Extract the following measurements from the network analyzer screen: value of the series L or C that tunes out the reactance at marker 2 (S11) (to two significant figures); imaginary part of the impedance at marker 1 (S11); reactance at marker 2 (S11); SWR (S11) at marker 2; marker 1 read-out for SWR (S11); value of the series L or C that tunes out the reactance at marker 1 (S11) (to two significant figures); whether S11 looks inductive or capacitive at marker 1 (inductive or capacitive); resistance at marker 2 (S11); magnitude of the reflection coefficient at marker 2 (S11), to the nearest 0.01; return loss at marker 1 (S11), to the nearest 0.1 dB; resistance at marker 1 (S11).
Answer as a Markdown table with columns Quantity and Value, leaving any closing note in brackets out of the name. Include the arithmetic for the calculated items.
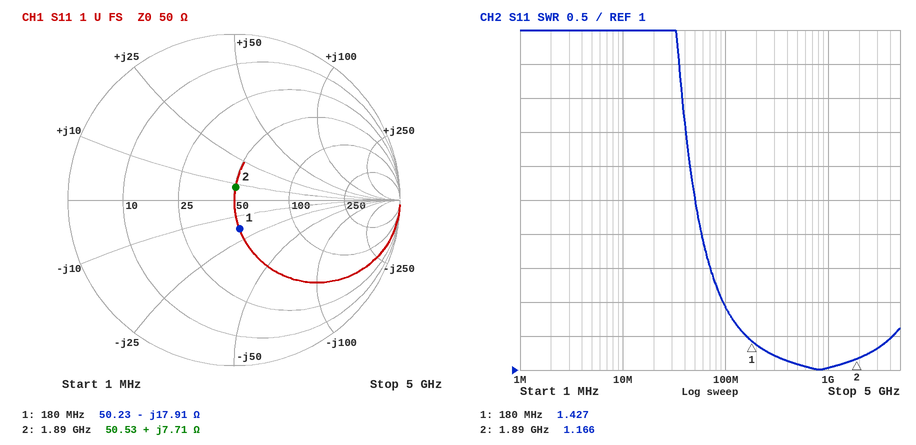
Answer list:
| Quantity | Value |
|---|---|
| value of the series L or C that tunes out the reactance at marker 2 (S11) | C = 1/(2π × 1.89 GHz × 7.71 Ω) ≈ 11 pF |
| imaginary part of the impedance at marker 1 | -17.91 Ω |
| reactance at marker 2 | +7.71 Ω |
| SWR (S11) at marker 2 | 1.166 |
| marker 1 read-out for SWR | 1.427 |
| value of the series L or C that tunes out the reactance at marker 1 (S11) | L = 17.91 Ω/(2π × 180 MHz) ≈ 16 nH |
| whether S11 looks inductive or capacitive at marker 1 | capacitive |
| resistance at marker 2 | 50.53 Ω |
| magnitude of the reflection coefficient at marker 2 (S11), to the nearest 0.01 | 0.08 |
| return loss at marker 1 (S11), to the nearest 0.1 dB | 15.1 dB |
| resistance at marker 1 | 50.23 Ω |
